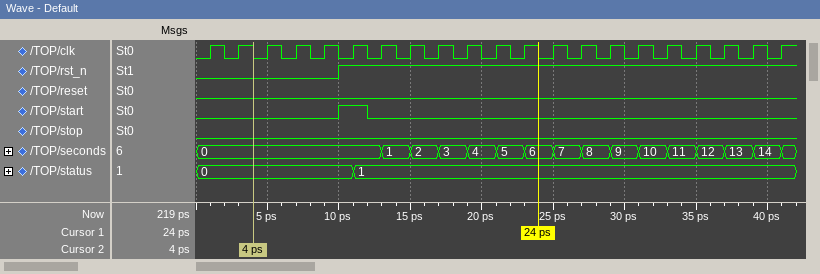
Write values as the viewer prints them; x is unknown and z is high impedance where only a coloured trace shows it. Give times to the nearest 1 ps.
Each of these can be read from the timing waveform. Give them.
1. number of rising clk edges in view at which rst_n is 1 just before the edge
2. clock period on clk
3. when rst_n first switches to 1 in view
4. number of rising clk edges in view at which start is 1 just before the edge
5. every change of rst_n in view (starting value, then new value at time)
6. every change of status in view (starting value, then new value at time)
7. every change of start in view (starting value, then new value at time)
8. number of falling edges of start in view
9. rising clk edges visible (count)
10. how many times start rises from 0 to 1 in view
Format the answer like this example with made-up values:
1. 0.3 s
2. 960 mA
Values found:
1. 16
2. 2 ps
3. 10 ps
4. 1
5. 0, 1 at 10 ps
6. 0, 1 at 11 ps
7. 0, 1 at 10 ps, 0 at 12 ps
8. 1
9. 21
10. 1
